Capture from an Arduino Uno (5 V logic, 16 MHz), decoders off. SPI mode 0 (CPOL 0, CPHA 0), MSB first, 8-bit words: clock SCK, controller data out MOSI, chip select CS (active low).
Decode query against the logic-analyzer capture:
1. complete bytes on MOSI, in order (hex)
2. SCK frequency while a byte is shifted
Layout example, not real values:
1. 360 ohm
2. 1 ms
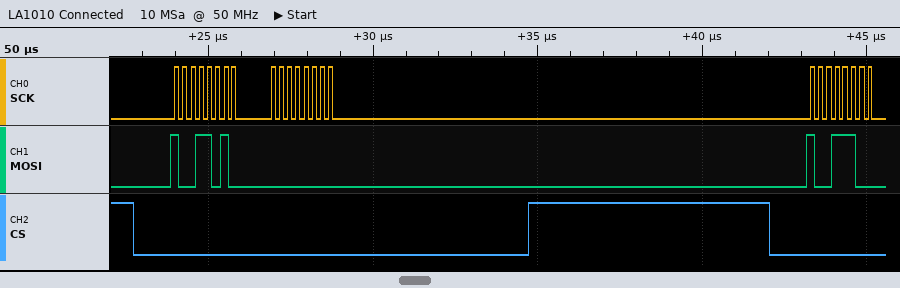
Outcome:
1. 9A 00 9C
2. 4 MHz
